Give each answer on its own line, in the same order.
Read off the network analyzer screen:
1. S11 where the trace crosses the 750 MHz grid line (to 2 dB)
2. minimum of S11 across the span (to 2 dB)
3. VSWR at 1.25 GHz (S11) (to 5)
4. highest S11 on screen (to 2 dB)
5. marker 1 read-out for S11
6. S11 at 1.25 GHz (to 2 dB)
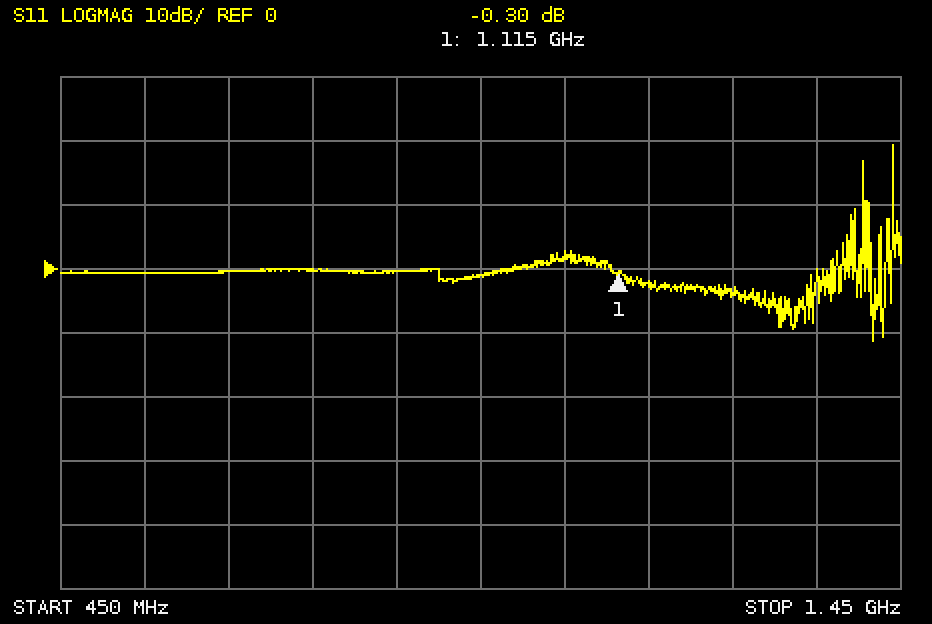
0 dB
-12 dB
5
20 dB
-0.30 dB
-4 dB
